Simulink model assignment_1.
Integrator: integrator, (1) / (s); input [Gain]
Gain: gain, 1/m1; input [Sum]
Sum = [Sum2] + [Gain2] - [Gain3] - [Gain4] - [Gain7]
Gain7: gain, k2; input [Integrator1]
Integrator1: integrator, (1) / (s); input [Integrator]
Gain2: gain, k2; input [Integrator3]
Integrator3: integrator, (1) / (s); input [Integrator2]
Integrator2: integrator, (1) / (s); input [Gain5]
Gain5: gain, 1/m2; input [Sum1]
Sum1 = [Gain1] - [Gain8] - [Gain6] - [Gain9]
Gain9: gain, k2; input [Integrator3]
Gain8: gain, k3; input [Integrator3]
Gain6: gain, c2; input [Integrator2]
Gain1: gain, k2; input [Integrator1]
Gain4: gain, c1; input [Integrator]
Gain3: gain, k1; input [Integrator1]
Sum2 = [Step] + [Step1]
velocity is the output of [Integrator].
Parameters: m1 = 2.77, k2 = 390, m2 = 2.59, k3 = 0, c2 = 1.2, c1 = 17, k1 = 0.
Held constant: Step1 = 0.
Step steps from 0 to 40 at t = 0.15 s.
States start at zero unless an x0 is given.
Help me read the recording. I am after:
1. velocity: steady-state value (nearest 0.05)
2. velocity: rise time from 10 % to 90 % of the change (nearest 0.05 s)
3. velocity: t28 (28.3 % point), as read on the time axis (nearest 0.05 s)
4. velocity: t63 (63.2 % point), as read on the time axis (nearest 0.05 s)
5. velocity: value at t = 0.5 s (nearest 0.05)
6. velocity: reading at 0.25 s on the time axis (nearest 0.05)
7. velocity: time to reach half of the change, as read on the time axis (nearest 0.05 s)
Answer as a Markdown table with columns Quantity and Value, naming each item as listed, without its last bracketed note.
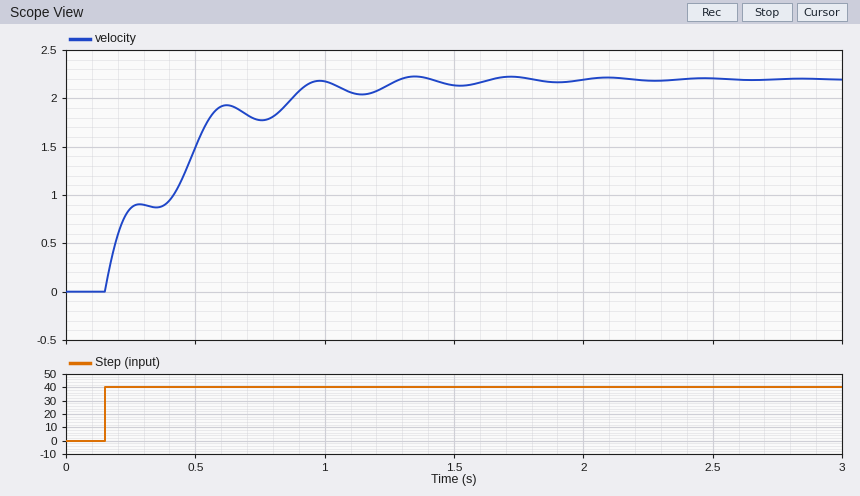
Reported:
| Quantity | Value |
|---|---|
| velocity: steady-state value | 2.20 |
| velocity: rise time from 10 % to 90 % of the change | 0.70 s |
| velocity: t28 (28.3 % point), as read on the time axis | 0.20 s |
| velocity: t63 (63.2 % point), as read on the time axis | 0.50 s |
| velocity: value at t = 0.5 s | 1.50 |
| velocity: reading at 0.25 s on the time axis | 0.85 |
| velocity: time to reach half of the change, as read on the time axis | 0.45 s |
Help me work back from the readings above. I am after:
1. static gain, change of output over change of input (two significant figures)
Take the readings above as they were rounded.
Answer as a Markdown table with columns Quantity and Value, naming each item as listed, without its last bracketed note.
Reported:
| Quantity | Value |
|---|---|
| static gain, change of output over change of input | 0.055 |
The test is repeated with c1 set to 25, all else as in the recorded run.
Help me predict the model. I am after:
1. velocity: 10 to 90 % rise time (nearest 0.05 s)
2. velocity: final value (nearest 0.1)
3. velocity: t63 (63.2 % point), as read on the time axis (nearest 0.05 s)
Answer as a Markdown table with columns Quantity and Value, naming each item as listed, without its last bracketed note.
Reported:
| Quantity | Value |
|---|---|
| velocity: 10 to 90 % rise time | 0.35 s |
| velocity: final value | 1.5 |
| velocity: t63 (63.2 % point), as read on the time axis | 0.45 s |
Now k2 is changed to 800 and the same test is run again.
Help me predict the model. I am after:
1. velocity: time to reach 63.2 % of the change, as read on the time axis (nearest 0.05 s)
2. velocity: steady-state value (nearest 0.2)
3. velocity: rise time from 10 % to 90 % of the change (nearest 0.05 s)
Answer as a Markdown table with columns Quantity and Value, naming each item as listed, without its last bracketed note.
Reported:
| Quantity | Value |
|---|---|
| velocity: time to reach 63.2 % of the change, as read on the time axis | 0.40 s |
| velocity: steady-state value | 2.2 |
| velocity: rise time from 10 % to 90 % of the change | 0.55 s |
